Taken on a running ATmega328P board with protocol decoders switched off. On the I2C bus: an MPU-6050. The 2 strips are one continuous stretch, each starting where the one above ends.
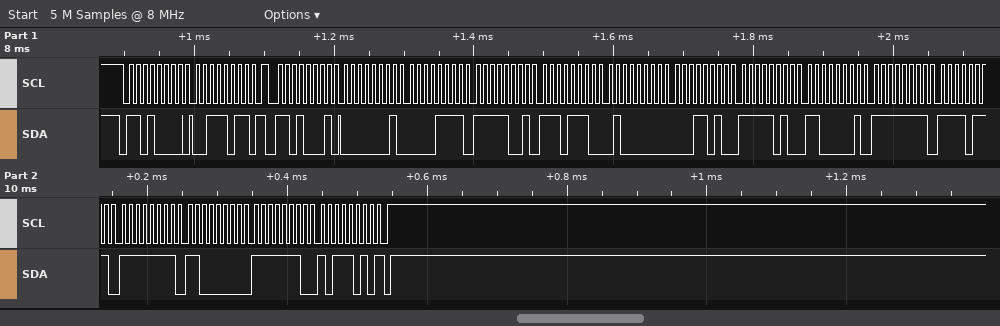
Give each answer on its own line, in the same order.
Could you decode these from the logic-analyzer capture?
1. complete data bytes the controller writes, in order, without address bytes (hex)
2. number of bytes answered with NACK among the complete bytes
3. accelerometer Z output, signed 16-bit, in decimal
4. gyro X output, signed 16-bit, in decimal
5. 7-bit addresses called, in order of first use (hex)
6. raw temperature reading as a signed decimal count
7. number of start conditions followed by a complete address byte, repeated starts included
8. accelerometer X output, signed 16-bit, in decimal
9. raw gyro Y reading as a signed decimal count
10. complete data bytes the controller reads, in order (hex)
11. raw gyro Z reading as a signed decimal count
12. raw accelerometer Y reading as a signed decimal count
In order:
3B
1
16410
-9
0x68
-1343
2
271
-64
01 0F F9 EE 40 1A FA C1 FF F7 FF C0 FE BA
-326
-1554
